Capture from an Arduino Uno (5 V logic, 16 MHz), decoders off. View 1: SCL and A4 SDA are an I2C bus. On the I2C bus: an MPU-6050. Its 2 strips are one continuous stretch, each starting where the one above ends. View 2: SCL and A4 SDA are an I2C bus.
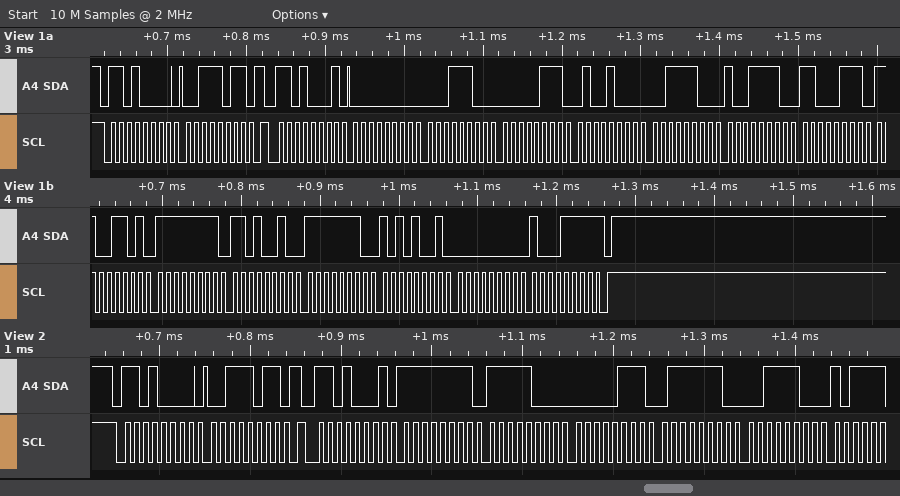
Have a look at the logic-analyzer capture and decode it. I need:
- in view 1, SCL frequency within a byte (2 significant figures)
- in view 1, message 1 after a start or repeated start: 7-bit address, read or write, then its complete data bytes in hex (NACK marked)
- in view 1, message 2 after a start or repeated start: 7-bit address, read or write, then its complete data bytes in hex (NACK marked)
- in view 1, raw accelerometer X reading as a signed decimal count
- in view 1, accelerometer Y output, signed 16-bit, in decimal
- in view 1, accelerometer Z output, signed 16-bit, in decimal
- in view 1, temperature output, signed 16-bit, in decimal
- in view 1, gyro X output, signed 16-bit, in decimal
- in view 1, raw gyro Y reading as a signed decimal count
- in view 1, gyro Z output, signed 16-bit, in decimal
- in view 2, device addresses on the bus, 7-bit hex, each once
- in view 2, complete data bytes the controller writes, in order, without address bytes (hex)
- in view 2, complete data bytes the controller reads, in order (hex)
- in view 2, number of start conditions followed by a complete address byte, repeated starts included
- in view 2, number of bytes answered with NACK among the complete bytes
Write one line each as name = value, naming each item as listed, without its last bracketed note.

in view 1, SCL frequency within a byte = 100 kHz
in view 1, message 1 after a start or repeated start: 7-bit address, read or write, then its complete data bytes in hex = 0x68 write: 3B
in view 1, message 2 after a start or repeated start: 7-bit address, read or write, then its complete data bytes in hex = 0x68 read: 00 1C 07 48 3C 9E C7 CD FF D2 FE A9 00 8F NACK
in view 1, raw accelerometer X reading as a signed decimal count = 28
in view 1, accelerometer Y output, signed 16-bit, in decimal = 1864
in view 1, accelerometer Z output, signed 16-bit, in decimal = 15518
in view 1, temperature output, signed 16-bit, in decimal = -14387
in view 1, gyro X output, signed 16-bit, in decimal = -46
in view 1, raw gyro Y reading as a signed decimal count = -343
in view 1, gyro Z output, signed 16-bit, in decimal = 143
in view 2, device addresses on the bus, 7-bit hex, each once = 0x68
in view 2, complete data bytes the controller writes, in order, without address bytes = 3B
in view 2, complete data bytes the controller reads, in order = FF F8 07 7E 3C
in view 2, number of start conditions followed by a complete address byte, repeated starts included = 2
in view 2, number of bytes answered with NACK among the complete bytes = 0
